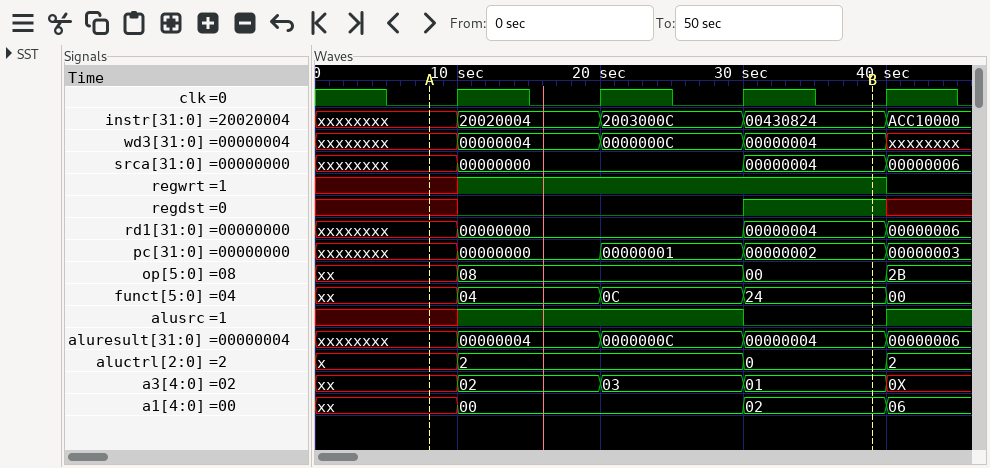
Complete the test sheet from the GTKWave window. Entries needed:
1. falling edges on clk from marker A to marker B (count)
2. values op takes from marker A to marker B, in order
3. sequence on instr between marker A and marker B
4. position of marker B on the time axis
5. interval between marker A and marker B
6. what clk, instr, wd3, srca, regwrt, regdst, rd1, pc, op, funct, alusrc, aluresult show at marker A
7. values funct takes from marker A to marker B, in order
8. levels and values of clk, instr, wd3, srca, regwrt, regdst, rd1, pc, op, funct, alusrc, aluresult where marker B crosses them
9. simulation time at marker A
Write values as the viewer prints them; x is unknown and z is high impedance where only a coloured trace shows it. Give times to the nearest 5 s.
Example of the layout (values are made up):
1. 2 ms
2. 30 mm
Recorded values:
1. 3
2. xx, 08, 00
3. xxxxxxxx, 20020004, 2003000C, 00430824
4. 40 s
5. 30 s
6. clk=0, instr=xxxxxxxx, wd3=xxxxxxxx, srca=xxxxxxxx, regwrt=x, regdst=x, rd1=xxxxxxxx, pc=xxxxxxxx, op=xx, funct=xx, alusrc=x, aluresult=xxxxxxxx
7. xx, 04, 0C, 24
8. clk=0, instr=00430824, wd3=00000004, srca=00000004, regwrt=1, regdst=1, rd1=00000004, pc=00000002, op=00, funct=24, alusrc=0, aluresult=00000004
9. 10 s
